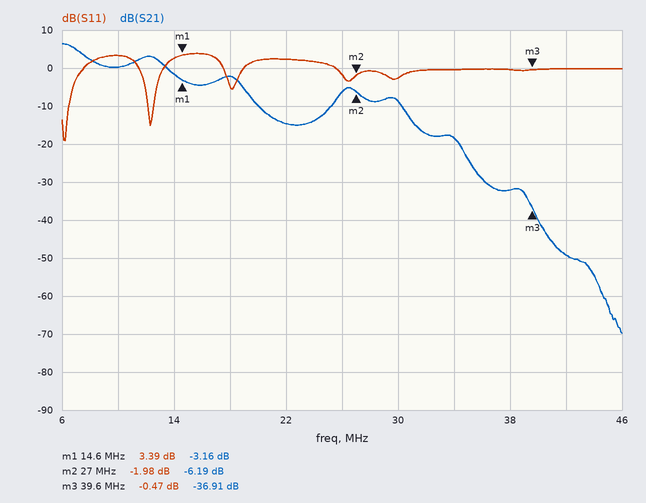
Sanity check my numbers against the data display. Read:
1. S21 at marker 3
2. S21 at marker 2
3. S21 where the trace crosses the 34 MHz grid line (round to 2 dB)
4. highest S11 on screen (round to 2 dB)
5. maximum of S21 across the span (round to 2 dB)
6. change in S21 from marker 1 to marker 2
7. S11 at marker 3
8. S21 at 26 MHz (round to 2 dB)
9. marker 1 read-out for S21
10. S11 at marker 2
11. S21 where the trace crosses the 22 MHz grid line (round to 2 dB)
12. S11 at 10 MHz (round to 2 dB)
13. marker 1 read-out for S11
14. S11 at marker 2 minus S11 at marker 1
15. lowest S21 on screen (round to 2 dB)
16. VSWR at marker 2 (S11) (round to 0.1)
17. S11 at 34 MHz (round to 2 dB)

-36.91 dB
-6.19 dB
-18 dB
4 dB
6 dB
-3.03 dB
-0.47 dB
-6 dB
-3.16 dB
-1.98 dB
-14 dB
4 dB
3.39 dB
-5.37 dB
-70 dB
8.8
0 dB
